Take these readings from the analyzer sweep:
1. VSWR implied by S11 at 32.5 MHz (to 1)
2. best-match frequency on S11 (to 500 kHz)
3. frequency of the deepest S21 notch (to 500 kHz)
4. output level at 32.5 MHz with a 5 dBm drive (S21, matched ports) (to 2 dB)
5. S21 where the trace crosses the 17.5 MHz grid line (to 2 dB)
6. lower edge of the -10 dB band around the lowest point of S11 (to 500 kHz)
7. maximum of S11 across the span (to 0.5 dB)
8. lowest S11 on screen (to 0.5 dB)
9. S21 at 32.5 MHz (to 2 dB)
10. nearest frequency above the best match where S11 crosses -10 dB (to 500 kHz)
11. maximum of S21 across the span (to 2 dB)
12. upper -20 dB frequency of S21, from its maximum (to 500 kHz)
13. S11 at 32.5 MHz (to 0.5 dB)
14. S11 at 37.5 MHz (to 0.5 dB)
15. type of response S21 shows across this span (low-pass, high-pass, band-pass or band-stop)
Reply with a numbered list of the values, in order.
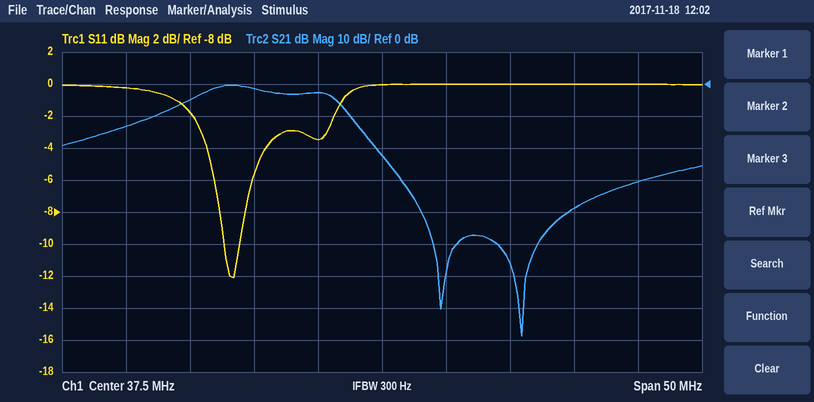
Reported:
1. 5
2. 26.0 MHz
3. 48.5 MHz
4. 2 dBm
5. -14 dB
6. 25.0 MHz
7. 0.0 dB
8. -12.0 dB
9. -2 dB
10. 26.5 MHz
11. 0 dB
12. 37.0 MHz
13. -3.5 dB
14. 0.0 dB
15. band-pass
